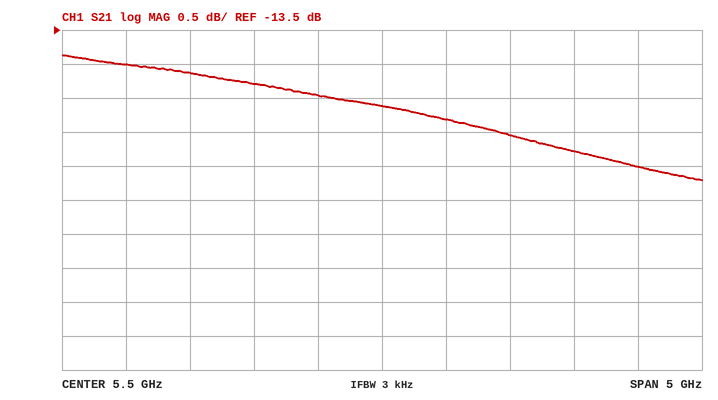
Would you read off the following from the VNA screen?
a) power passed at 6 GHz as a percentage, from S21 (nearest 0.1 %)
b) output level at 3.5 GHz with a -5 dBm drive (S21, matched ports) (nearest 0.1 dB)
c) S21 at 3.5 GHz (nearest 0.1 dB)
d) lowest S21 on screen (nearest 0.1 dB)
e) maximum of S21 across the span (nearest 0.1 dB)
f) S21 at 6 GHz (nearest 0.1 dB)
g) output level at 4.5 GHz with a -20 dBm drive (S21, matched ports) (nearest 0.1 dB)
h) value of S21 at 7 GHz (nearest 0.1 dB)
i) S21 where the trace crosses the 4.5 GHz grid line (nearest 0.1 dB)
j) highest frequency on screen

3.3 %
-19.0 dBm
-14.0 dB
-15.7 dB
-13.9 dB
-14.8 dB
-34.3 dBm
-15.3 dB
-14.3 dB
8 GHz
